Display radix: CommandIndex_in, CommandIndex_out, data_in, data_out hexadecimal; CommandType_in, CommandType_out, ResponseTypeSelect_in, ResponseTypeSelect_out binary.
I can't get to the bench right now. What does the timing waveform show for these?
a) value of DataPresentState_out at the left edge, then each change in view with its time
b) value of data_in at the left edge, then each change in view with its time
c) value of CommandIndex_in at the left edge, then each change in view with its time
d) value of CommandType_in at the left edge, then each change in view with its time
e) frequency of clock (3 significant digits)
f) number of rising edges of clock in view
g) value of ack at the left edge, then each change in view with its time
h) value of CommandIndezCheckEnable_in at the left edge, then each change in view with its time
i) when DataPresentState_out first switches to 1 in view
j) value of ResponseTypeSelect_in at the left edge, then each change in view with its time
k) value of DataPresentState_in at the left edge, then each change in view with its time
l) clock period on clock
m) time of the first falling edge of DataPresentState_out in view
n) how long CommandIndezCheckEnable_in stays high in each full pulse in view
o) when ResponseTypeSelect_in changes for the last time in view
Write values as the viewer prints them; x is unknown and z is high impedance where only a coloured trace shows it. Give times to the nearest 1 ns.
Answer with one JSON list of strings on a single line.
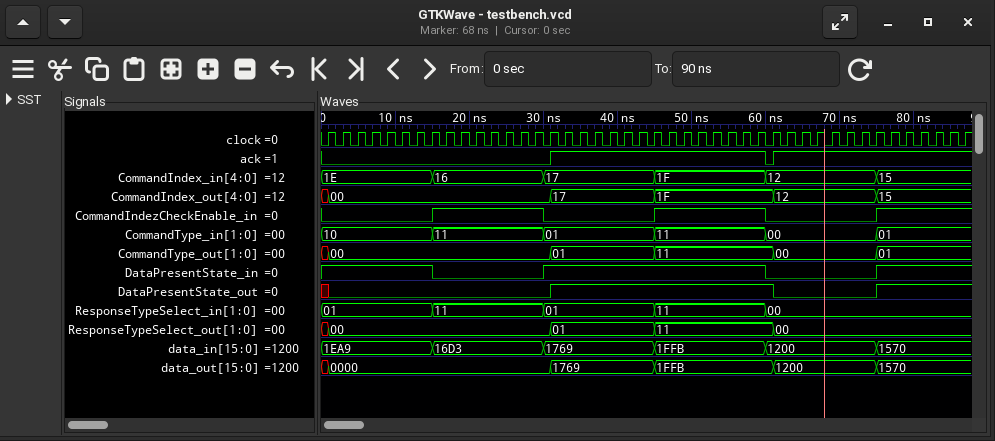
["x, 0 at 1 ns, 1 at 31 ns, 0 at 61 ns, 1 at 75 ns", "1EA9, 16D3 at 15 ns, 1769 at 30 ns, 1FFB at 45 ns, 1200 at 60 ns, 1570 at 75 ns", "1E, 16 at 15 ns, 17 at 30 ns, 1F at 45 ns, 12 at 60 ns, 15 at 75 ns", "10, 11 at 15 ns, 01 at 30 ns, 11 at 45 ns, 00 at 60 ns, 01 at 75 ns", "500 MHz", "44", "0, 1 at 31 ns, 0 at 60 ns, 1 at 61 ns", "0, 1 at 15 ns, 0 at 30 ns, 1 at 45 ns, 0 at 60 ns, 1 at 75 ns", "31 ns", "01, 11 at 15 ns, 01 at 30 ns, 11 at 45 ns, 00 at 60 ns", "1, 0 at 15 ns, 1 at 30 ns, 0 at 60 ns, 1 at 75 ns", "2 ns", "61 ns", "15 ns, 15 ns", "60 ns"]
